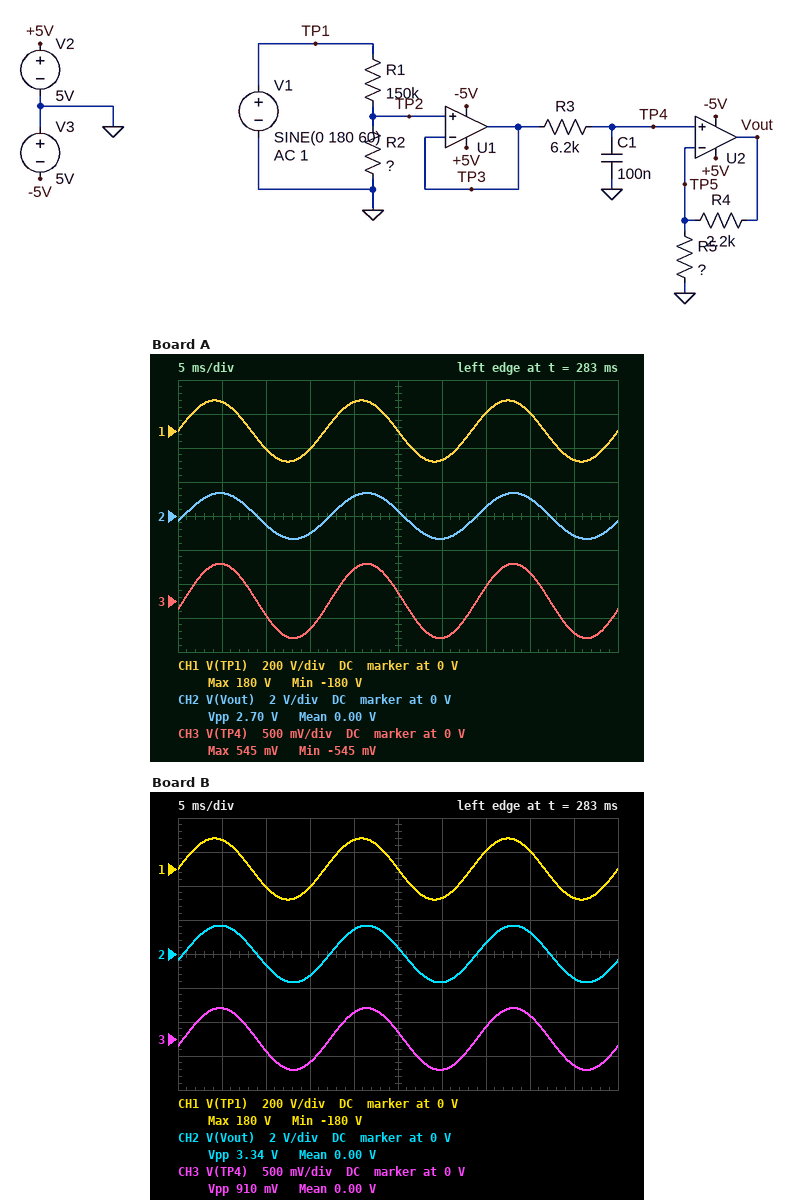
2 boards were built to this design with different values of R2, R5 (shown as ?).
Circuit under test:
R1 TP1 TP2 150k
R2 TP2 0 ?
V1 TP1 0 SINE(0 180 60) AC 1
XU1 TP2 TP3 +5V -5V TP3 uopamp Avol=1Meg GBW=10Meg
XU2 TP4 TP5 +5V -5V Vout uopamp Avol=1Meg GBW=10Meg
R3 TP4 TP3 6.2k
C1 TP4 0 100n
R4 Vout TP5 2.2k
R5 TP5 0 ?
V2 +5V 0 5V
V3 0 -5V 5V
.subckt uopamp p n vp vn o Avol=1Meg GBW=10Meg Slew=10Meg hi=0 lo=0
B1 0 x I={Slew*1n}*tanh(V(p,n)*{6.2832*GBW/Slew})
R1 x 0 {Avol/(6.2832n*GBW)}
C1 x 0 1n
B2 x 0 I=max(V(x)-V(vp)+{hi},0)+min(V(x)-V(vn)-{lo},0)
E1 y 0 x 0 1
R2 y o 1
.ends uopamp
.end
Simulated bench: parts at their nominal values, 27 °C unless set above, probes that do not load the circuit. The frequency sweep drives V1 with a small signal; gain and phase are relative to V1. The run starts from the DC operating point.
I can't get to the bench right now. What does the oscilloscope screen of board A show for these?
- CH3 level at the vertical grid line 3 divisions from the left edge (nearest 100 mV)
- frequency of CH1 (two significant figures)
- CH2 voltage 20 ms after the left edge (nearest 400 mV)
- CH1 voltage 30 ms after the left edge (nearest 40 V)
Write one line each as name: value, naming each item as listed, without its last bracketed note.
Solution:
CH3 level at the vertical grid line 3 divisions from the left edge: -400 mV
frequency of CH1: 60 Hz
CH2 voltage 20 ms after the left edge: 1.2 V
CH1 voltage 30 ms after the left edge: -160 V
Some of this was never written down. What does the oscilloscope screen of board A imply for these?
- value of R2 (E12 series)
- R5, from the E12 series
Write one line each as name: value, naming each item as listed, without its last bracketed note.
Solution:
value of R2: 470 Ω
R5, from the E12 series: 1.5 kΩ
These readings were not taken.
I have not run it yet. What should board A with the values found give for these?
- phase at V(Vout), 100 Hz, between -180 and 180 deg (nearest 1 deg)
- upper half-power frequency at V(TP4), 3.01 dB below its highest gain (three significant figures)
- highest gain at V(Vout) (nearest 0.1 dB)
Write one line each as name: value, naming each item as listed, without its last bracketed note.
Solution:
phase at V(Vout), 100 Hz, between -180 and 180 deg: -21 deg
upper half-power frequency at V(TP4), 3.01 dB below its highest gain: 257 Hz
highest gain at V(Vout): -42.3 dB
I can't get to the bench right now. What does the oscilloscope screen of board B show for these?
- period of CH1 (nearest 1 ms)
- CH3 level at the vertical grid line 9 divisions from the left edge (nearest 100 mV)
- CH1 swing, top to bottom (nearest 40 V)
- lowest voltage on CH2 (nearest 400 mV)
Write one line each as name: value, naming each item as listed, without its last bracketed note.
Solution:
period of CH1: 17 ms
CH3 level at the vertical grid line 9 divisions from the left edge: -400 mV
CH1 swing, top to bottom: 360 V
lowest voltage on CH2: -1.6 V
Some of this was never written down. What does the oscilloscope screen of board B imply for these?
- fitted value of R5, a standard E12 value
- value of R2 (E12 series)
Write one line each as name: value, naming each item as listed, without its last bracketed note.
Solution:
fitted value of R5, a standard E12 value: 820 Ω
value of R2: 390 Ω
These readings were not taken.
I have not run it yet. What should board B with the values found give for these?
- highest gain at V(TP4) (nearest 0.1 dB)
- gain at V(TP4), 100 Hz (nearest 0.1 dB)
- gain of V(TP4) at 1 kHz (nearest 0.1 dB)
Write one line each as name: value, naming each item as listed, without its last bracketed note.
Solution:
highest gain at V(TP4): -51.7 dB
gain at V(TP4), 100 Hz: -52.3 dB
gain of V(TP4) at 1 kHz: -63.8 dB
